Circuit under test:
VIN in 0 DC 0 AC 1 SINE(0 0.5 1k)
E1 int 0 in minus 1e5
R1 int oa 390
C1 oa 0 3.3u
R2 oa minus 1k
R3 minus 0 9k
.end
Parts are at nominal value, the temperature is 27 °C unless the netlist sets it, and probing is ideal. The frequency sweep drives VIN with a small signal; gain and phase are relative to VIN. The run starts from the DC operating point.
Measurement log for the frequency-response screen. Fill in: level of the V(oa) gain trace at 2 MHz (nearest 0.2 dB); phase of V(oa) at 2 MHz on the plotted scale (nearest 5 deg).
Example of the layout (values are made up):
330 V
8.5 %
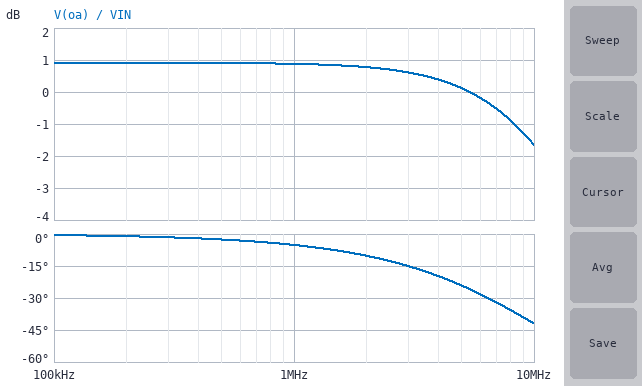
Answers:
0.8 dB
-10 deg
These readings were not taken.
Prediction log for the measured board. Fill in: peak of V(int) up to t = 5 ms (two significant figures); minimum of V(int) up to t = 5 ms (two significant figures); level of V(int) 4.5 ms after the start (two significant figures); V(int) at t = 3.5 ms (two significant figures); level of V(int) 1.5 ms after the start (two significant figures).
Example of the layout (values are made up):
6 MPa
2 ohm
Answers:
4.5 V
-4.5 V
-4.5 V
-4.5 V
-4.5 V
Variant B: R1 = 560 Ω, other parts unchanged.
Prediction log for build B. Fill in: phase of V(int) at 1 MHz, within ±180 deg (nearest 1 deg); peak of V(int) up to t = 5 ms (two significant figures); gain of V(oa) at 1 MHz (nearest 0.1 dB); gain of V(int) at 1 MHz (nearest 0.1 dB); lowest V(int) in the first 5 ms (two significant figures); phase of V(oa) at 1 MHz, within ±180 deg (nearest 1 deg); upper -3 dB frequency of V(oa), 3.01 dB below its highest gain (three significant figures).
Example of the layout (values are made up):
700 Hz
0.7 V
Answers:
83 deg
6.5 V
0.8 dB
82.1 dB
-6.5 V
-7 deg
7.75 MHz
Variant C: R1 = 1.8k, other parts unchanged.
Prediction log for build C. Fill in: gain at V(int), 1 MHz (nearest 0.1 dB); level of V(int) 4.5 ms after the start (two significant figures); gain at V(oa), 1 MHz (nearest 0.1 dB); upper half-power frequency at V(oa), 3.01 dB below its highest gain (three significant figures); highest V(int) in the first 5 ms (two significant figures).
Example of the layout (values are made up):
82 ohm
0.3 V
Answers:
91.7 dB
-21 V
0.2 dB
2.41 MHz
21 V
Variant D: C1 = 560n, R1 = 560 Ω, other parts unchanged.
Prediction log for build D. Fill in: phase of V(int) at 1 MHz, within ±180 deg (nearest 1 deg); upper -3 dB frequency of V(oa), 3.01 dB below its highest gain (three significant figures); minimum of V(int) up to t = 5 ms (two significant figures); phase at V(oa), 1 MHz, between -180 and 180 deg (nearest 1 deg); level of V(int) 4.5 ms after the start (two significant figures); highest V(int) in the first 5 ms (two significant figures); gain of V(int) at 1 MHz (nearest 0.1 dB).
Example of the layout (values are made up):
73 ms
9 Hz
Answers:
89 deg
45.7 MHz
-1.2 V
-1 deg
-1.1 V
1.2 V
66.8 dB
